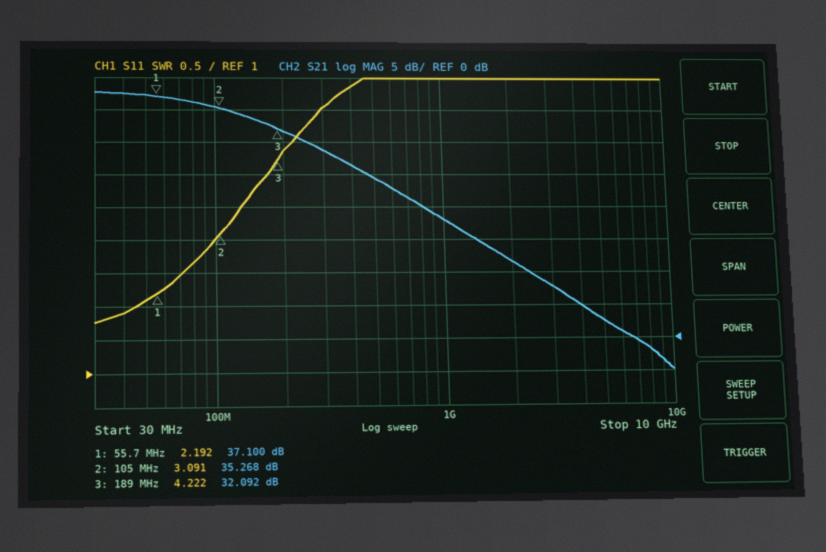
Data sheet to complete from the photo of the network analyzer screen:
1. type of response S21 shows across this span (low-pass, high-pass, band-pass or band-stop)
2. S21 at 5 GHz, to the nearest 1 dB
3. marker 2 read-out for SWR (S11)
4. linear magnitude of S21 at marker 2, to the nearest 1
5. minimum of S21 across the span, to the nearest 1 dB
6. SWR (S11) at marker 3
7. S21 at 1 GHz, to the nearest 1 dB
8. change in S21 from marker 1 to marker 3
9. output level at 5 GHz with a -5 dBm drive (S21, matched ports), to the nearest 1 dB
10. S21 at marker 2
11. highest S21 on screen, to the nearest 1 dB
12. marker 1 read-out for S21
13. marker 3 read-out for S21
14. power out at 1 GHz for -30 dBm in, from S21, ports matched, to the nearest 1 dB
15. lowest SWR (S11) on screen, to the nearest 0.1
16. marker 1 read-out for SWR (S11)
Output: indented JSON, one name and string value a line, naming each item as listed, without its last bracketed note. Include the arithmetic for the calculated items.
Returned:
{
  "type of response S21 shows across this span": "low-pass",
  "S21 at 5 GHz, to the nearest 1 dB": "3 dB",
  "marker 2 read-out for SWR": "3.091",
  "linear magnitude of S21 at marker 2, to the nearest 1": "10^(35.268/20) ≈ 58",
  "minimum of S21 across the span, to the nearest 1 dB": "-5 dB",
  "SWR (S11) at marker 3": "4.222",
  "S21 at 1 GHz, to the nearest 1 dB": "18 dB",
  "change in S21 from marker 1 to marker 3": "32.092 − (37.1) = -5.008 dB",
  "output level at 5 GHz with a -5 dBm drive (S21, matched ports), to the nearest 1 dB": "-5 dBm + (3 dB) = -2 dBm",
  "S21 at marker 2": "35.268 dB",
  "highest S21 on screen, to the nearest 1 dB": "38 dB",
  "marker 1 read-out for S21": "37.100 dB",
  "marker 3 read-out for S21": "32.092 dB",
  "power out at 1 GHz for -30 dBm in, from S21, ports matched, to the nearest 1 dB": "-30 dBm + (18 dB) = -12 dBm",
  "lowest SWR (S11) on screen, to the nearest 0.1": "1.8",
  "marker 1 read-out for SWR": "2.192"
}
